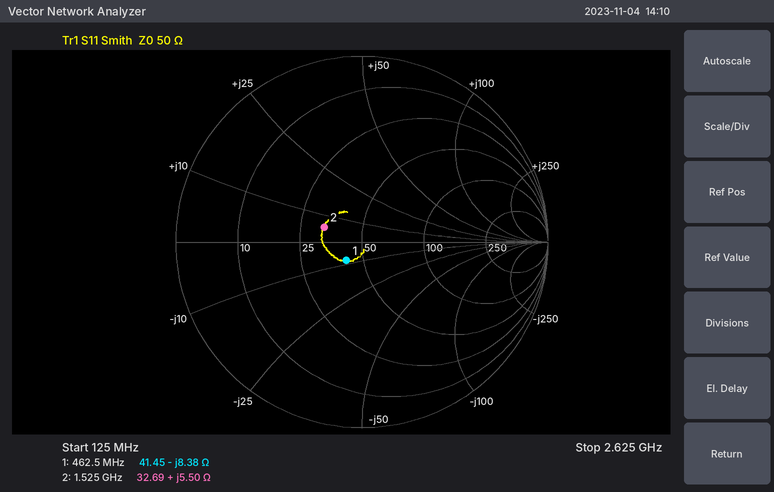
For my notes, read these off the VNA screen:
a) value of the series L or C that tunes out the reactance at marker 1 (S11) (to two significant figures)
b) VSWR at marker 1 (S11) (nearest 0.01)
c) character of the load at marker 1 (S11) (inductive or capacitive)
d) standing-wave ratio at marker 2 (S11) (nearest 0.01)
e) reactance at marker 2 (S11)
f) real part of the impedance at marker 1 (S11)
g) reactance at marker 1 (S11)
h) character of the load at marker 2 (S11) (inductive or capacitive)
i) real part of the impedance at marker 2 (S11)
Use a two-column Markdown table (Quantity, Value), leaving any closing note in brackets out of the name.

| Quantity | Value |
|---|---|
| value of the series L or C that tunes out the reactance at marker 1 (S11) | 2.9 nH |
| VSWR at marker 1 (S11) | 1.30 |
| character of the load at marker 1 (S11) | capacitive |
| standing-wave ratio at marker 2 (S11) | 1.56 |
| reactance at marker 2 | +5.50 Ω |
| real part of the impedance at marker 1 | 41.45 Ω |
| reactance at marker 1 | -8.38 Ω |
| character of the load at marker 2 (S11) | inductive |
| real part of the impedance at marker 2 | 32.69 Ω |
